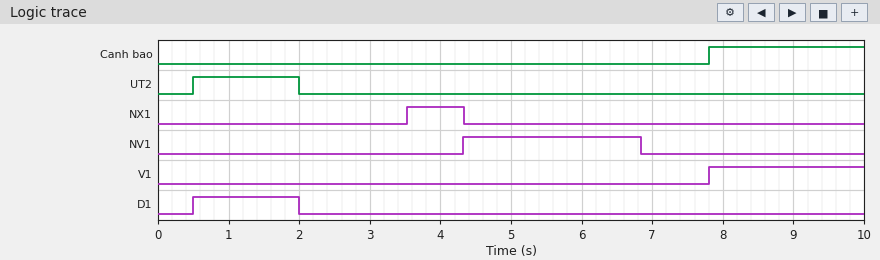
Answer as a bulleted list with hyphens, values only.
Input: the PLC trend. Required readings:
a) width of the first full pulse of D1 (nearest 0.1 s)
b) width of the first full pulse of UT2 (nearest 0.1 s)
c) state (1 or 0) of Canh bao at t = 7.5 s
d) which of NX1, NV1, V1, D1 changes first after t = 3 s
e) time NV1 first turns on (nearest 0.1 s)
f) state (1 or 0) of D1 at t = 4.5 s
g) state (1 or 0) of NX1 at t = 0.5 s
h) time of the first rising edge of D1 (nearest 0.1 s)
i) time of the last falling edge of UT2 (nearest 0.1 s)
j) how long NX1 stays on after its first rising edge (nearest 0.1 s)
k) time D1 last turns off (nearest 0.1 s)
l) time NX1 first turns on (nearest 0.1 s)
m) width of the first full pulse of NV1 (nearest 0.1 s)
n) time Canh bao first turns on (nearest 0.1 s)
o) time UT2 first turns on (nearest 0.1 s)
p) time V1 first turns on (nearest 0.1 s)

- 1.5 s
- 1.5 s
- 0
- NX1
- 4.3 s
- 0
- 0
- 0.5 s
- 2.0 s
- 0.8 s
- 2.0 s
- 3.5 s
- 2.5 s
- 7.8 s
- 0.5 s
- 7.8 s
